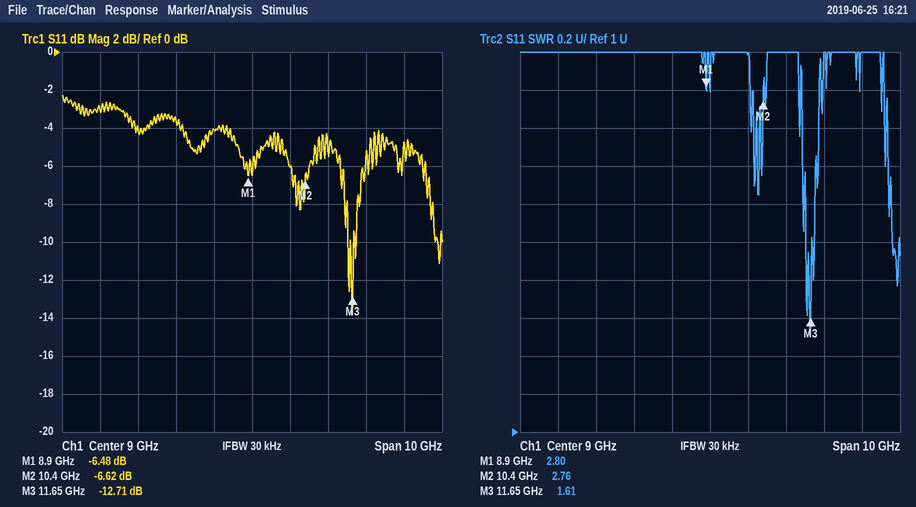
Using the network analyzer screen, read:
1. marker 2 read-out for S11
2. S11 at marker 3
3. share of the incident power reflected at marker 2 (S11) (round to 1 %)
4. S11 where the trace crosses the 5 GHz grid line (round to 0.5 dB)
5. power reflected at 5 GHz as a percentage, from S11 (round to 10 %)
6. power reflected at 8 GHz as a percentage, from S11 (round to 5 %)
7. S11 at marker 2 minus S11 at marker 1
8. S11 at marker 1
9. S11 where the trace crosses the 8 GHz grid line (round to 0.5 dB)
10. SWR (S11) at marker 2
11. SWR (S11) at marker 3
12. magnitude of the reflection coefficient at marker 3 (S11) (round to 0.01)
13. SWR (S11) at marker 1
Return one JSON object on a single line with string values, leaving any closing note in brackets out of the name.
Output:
{"marker 2 read-out for S11": "-6.62 dB", "S11 at marker 3": "-12.71 dB", "share of the incident power reflected at marker 2 (S11)": "22 %", "S11 where the trace crosses the 5 GHz grid line": "-3.0 dB", "power reflected at 5 GHz as a percentage, from S11": "50 %", "power reflected at 8 GHz as a percentage, from S11": "40 %", "S11 at marker 2 minus S11 at marker 1": "-0.14 dB", "S11 at marker 1": "-6.48 dB", "S11 where the trace crosses the 8 GHz grid line": "-4.0 dB", "SWR (S11) at marker 2": "2.76", "SWR (S11) at marker 3": "1.61", "magnitude of the reflection coefficient at marker 3 (S11)": "0.23", "SWR (S11) at marker 1": "2.80"}
